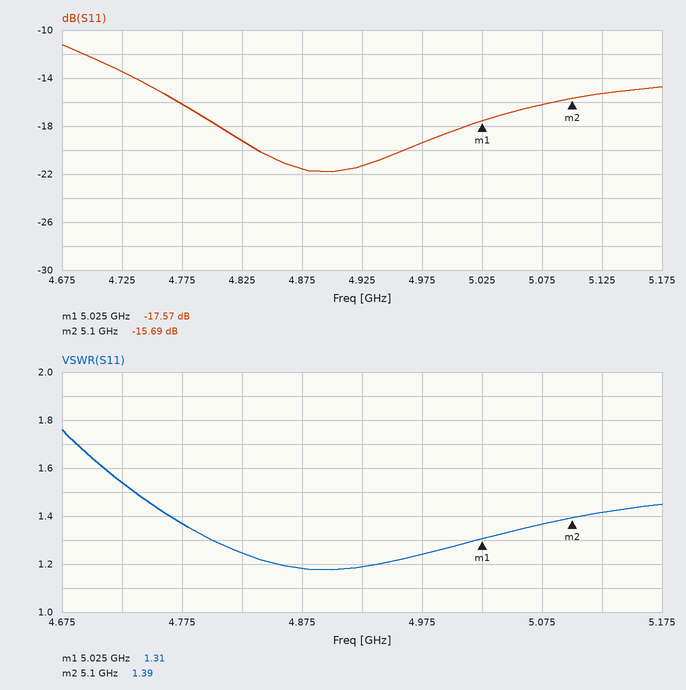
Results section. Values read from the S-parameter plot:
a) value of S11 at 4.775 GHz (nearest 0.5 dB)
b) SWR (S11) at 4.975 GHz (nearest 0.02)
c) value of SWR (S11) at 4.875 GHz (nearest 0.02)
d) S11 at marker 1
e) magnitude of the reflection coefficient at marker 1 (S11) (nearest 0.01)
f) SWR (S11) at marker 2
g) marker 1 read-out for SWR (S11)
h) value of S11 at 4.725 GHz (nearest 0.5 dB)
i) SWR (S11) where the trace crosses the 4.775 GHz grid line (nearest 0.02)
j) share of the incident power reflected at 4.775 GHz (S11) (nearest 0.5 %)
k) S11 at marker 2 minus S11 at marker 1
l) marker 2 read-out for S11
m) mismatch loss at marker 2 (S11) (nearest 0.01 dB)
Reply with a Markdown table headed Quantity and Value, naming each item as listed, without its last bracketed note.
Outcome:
| Quantity | Value |
|---|---|
| value of S11 at 4.775 GHz | -16.0 dB |
| SWR (S11) at 4.975 GHz | 1.24 |
| value of SWR (S11) at 4.875 GHz | 1.18 |
| S11 at marker 1 | -17.57 dB |
| magnitude of the reflection coefficient at marker 1 (S11) | 0.13 |
| SWR (S11) at marker 2 | 1.39 |
| marker 1 read-out for SWR | 1.31 |
| value of S11 at 4.725 GHz | -13.5 dB |
| SWR (S11) where the trace crosses the 4.775 GHz grid line | 1.36 |
| share of the incident power reflected at 4.775 GHz (S11) | 2.5 % |
| S11 at marker 2 minus S11 at marker 1 | 1.88 dB |
| marker 2 read-out for S11 | -15.69 dB |
| mismatch loss at marker 2 (S11) | 0.12 dB |
